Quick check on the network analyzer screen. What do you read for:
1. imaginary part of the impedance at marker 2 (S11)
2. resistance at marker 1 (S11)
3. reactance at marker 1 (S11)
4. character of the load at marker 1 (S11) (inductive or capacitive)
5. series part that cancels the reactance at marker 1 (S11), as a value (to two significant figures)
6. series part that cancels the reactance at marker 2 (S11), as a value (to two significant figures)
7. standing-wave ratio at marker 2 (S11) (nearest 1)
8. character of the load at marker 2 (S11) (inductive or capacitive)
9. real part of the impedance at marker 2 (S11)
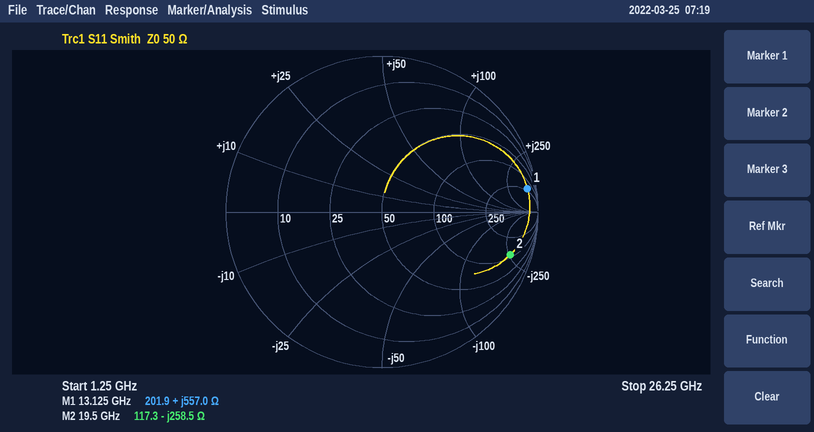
-258.5 Ω
201.9 Ω
+557.0 Ω
inductive
22 fF
2.1 nH
14
capacitive
117.3 Ω
